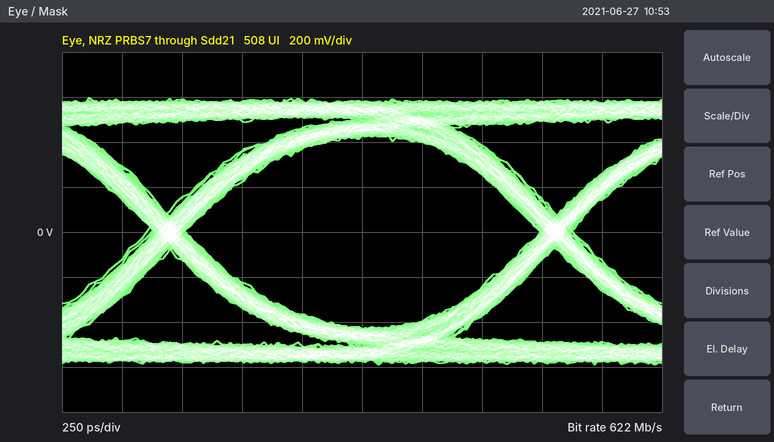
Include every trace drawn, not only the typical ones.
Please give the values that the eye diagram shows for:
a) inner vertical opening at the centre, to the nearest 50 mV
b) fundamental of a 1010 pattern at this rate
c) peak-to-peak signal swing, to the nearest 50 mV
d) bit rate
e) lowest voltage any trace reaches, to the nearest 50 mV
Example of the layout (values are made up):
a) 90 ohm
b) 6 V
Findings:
a) 850 mV
b) 311 MHz
c) 1.20 V
d) 622 Mb/s
e) -600 mV
